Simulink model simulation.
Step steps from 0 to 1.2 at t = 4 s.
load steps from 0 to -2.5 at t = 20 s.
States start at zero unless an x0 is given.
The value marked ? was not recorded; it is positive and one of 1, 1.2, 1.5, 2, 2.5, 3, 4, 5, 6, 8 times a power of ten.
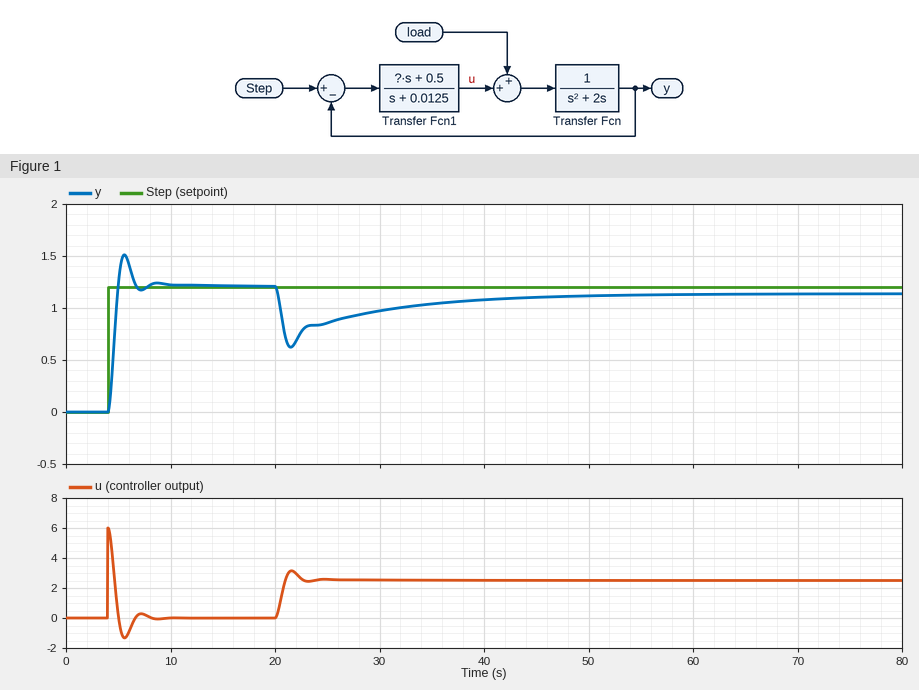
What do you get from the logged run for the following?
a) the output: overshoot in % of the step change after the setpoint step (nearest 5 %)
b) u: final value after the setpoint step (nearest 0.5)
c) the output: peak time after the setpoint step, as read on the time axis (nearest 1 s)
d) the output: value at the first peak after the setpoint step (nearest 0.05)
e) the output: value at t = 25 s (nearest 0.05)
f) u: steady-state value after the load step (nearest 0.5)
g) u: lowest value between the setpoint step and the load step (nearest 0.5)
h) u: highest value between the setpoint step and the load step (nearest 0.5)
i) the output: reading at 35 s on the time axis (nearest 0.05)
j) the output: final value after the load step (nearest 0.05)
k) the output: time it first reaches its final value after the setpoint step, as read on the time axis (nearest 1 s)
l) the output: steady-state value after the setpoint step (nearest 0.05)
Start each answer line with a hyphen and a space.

- 25 %
- 0.0
- 6 s
- 1.50
- 0.85
- 2.5
- -1.5
- 6.0
- 1.05
- 1.15
- 5 s
- 1.20
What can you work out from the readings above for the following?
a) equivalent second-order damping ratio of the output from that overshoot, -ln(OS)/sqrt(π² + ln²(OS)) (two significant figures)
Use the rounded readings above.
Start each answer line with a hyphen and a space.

- 0.40
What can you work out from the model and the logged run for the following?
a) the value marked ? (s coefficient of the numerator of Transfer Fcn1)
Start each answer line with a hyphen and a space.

- 5
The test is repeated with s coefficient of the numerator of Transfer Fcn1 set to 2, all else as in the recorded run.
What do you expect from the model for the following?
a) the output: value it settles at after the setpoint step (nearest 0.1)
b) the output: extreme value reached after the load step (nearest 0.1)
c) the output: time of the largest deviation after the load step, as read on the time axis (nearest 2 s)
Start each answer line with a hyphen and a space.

- 1.2
- 0.1
- 22 s
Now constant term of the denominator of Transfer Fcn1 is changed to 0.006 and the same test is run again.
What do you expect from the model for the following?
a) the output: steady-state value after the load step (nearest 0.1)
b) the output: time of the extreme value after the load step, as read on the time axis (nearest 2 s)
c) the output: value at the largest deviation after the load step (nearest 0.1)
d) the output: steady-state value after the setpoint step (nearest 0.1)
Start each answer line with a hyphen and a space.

- 1.2
- 22 s
- 0.6
- 1.2
